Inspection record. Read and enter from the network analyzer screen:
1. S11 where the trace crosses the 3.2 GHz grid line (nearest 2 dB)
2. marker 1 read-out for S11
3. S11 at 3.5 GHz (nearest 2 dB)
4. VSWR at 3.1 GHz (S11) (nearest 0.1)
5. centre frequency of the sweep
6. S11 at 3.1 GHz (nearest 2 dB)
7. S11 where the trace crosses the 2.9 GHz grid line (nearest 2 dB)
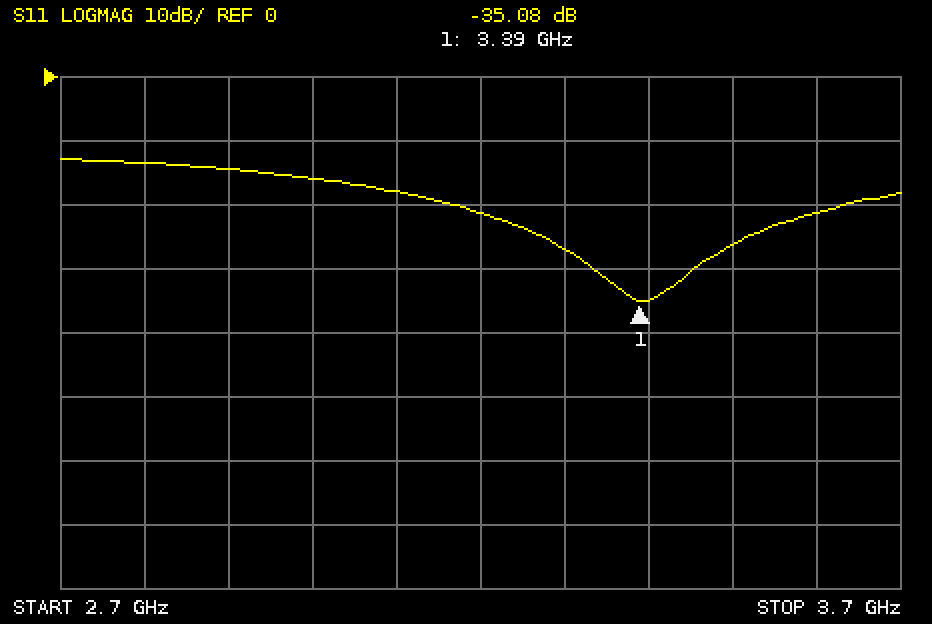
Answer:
-22 dB
-35.08 dB
-26 dB
1.3
3.2 GHz
-18 dB
-14 dB
